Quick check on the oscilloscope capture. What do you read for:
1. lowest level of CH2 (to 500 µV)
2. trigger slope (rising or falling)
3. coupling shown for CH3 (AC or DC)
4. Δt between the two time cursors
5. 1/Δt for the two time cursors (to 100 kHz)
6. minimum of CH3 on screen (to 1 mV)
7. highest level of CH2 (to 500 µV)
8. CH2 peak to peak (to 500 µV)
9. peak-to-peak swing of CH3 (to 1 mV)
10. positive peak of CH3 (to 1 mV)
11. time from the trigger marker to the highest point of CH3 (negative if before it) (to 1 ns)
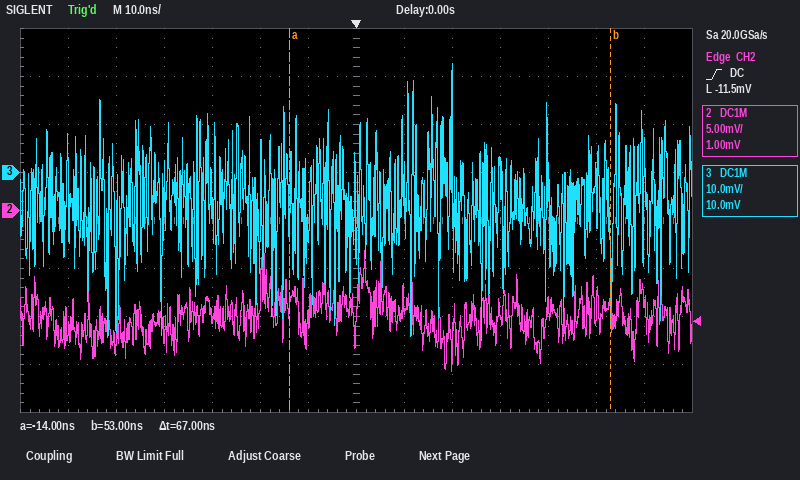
-16.5 mV
rising
DC
67 ns
14.9 MHz
-35 mV
-4.0 mV
12.5 mV
58 mV
23 mV
+20 ns
